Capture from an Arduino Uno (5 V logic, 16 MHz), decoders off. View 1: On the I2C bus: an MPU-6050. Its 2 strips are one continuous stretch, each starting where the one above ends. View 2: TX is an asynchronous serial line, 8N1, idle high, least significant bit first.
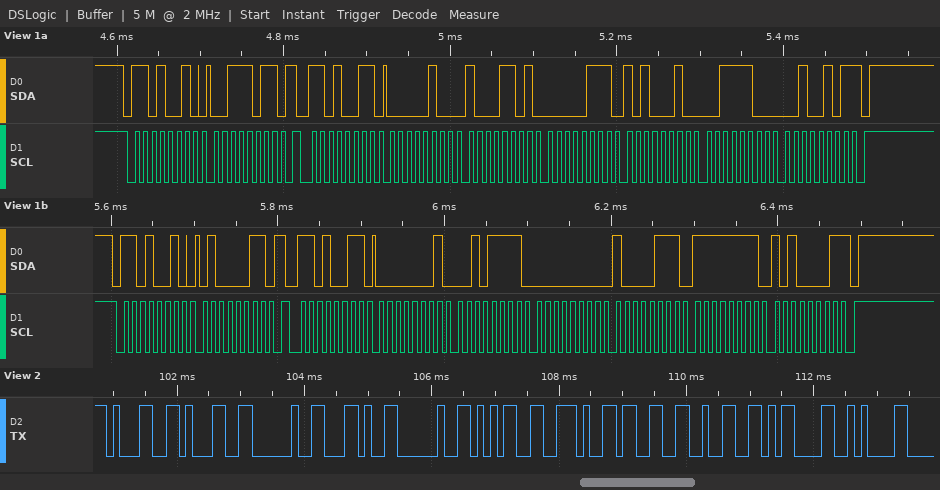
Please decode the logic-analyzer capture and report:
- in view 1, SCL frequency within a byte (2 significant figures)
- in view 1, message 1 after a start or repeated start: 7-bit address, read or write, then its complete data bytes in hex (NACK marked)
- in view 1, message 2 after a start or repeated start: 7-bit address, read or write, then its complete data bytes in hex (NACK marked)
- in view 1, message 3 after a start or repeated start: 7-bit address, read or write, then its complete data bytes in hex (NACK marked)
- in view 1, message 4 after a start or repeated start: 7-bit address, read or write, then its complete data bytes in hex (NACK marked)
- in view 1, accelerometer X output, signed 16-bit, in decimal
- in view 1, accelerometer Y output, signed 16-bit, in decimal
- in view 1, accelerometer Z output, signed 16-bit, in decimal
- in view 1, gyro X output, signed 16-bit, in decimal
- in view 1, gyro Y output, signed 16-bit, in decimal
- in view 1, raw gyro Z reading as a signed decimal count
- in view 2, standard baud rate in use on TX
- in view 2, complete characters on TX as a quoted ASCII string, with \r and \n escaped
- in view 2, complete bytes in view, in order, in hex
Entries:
100 kHz
0x69 write: 3B
0x69 read: 04 8D 07 A2 3C 25 NACK
0x69 write: 43
0x69 read: 01 2F 00 87 FF A1 NACK
1165
1954
15397
303
135
-95
9600 baud
"11 , 5.32\r\n"
0x31 0x31 0x20 0x2C 0x20 0x35 0x2E 0x33 0x32 0x0D 0x0A
